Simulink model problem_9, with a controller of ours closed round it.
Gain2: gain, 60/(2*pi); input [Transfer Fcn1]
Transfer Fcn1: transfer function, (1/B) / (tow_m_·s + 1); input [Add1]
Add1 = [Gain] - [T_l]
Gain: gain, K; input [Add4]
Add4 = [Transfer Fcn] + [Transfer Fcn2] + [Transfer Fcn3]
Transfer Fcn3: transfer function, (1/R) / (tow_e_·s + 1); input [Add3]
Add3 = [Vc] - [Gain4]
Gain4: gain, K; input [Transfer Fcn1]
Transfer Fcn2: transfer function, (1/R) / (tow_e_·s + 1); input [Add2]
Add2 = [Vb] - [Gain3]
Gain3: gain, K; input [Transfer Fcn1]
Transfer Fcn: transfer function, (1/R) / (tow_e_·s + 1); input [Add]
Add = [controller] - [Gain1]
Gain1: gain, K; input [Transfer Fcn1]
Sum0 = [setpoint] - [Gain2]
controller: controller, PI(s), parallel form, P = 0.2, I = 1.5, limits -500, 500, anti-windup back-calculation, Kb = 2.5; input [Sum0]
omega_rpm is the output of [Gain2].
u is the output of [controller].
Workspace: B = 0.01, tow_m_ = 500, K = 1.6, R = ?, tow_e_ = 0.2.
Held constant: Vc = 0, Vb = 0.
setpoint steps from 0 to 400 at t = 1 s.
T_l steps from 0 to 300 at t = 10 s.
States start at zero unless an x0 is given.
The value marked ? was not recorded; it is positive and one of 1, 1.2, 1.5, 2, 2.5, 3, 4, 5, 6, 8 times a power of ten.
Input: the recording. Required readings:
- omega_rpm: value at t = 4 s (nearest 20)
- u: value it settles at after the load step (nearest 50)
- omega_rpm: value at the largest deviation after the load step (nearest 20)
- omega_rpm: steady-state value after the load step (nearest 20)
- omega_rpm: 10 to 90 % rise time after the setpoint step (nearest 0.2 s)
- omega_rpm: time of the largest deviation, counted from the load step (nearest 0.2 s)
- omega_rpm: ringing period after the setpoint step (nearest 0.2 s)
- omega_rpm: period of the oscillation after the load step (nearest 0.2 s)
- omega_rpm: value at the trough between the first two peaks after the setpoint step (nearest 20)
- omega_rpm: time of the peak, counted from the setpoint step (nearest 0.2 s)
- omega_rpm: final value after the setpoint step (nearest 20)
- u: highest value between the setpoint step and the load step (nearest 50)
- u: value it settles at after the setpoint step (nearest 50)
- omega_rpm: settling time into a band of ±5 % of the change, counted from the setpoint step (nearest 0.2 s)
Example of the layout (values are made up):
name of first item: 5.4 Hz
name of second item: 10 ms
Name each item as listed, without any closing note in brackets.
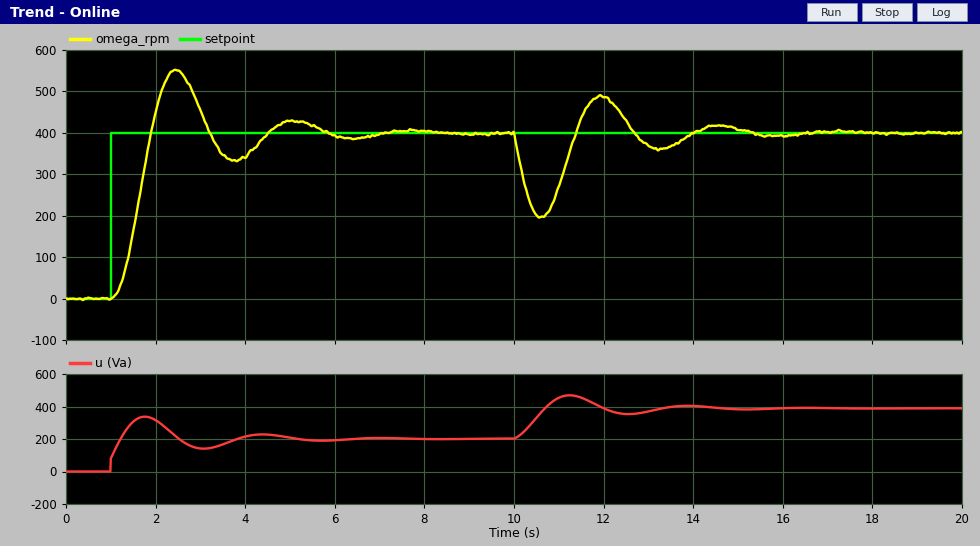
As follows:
omega_rpm: value at t = 4 s: 340
u: value it settles at after the load step: 400
omega_rpm: value at the largest deviation after the load step: 200
omega_rpm: steady-state value after the load step: 400
omega_rpm: 10 to 90 % rise time after the setpoint step: 0.6 s
omega_rpm: time of the largest deviation, counted from the load step: 0.6 s
omega_rpm: ringing period after the setpoint step: 2.6 s
omega_rpm: period of the oscillation after the load step: 2.6 s
omega_rpm: value at the trough between the first two peaks after the setpoint step: 340
omega_rpm: time of the peak, counted from the setpoint step: 1.4 s
omega_rpm: final value after the setpoint step: 400
u: highest value between the setpoint step and the load step: 350
u: value it settles at after the setpoint step: 200
omega_rpm: settling time into a band of ±5 % of the change, counted from the setpoint step: 4.4 s
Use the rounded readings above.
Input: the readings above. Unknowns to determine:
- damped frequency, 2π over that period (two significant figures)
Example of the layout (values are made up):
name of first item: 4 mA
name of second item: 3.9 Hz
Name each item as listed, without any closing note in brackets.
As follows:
damped frequency, 2π over that period: 2.4 rad/s
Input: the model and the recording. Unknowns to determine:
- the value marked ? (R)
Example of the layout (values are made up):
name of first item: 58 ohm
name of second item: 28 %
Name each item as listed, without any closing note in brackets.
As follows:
the value marked ?: 1
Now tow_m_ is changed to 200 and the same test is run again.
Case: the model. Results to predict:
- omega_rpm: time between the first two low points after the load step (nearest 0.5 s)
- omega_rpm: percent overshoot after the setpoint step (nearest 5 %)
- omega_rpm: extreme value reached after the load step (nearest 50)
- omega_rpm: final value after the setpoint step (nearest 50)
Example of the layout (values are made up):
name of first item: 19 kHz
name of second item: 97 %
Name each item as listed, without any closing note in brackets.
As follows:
omega_rpm: time between the first two low points after the load step: 1.5 s
omega_rpm: percent overshoot after the setpoint step: 20 %
omega_rpm: extreme value reached after the load step: 100
omega_rpm: final value after the setpoint step: 400
